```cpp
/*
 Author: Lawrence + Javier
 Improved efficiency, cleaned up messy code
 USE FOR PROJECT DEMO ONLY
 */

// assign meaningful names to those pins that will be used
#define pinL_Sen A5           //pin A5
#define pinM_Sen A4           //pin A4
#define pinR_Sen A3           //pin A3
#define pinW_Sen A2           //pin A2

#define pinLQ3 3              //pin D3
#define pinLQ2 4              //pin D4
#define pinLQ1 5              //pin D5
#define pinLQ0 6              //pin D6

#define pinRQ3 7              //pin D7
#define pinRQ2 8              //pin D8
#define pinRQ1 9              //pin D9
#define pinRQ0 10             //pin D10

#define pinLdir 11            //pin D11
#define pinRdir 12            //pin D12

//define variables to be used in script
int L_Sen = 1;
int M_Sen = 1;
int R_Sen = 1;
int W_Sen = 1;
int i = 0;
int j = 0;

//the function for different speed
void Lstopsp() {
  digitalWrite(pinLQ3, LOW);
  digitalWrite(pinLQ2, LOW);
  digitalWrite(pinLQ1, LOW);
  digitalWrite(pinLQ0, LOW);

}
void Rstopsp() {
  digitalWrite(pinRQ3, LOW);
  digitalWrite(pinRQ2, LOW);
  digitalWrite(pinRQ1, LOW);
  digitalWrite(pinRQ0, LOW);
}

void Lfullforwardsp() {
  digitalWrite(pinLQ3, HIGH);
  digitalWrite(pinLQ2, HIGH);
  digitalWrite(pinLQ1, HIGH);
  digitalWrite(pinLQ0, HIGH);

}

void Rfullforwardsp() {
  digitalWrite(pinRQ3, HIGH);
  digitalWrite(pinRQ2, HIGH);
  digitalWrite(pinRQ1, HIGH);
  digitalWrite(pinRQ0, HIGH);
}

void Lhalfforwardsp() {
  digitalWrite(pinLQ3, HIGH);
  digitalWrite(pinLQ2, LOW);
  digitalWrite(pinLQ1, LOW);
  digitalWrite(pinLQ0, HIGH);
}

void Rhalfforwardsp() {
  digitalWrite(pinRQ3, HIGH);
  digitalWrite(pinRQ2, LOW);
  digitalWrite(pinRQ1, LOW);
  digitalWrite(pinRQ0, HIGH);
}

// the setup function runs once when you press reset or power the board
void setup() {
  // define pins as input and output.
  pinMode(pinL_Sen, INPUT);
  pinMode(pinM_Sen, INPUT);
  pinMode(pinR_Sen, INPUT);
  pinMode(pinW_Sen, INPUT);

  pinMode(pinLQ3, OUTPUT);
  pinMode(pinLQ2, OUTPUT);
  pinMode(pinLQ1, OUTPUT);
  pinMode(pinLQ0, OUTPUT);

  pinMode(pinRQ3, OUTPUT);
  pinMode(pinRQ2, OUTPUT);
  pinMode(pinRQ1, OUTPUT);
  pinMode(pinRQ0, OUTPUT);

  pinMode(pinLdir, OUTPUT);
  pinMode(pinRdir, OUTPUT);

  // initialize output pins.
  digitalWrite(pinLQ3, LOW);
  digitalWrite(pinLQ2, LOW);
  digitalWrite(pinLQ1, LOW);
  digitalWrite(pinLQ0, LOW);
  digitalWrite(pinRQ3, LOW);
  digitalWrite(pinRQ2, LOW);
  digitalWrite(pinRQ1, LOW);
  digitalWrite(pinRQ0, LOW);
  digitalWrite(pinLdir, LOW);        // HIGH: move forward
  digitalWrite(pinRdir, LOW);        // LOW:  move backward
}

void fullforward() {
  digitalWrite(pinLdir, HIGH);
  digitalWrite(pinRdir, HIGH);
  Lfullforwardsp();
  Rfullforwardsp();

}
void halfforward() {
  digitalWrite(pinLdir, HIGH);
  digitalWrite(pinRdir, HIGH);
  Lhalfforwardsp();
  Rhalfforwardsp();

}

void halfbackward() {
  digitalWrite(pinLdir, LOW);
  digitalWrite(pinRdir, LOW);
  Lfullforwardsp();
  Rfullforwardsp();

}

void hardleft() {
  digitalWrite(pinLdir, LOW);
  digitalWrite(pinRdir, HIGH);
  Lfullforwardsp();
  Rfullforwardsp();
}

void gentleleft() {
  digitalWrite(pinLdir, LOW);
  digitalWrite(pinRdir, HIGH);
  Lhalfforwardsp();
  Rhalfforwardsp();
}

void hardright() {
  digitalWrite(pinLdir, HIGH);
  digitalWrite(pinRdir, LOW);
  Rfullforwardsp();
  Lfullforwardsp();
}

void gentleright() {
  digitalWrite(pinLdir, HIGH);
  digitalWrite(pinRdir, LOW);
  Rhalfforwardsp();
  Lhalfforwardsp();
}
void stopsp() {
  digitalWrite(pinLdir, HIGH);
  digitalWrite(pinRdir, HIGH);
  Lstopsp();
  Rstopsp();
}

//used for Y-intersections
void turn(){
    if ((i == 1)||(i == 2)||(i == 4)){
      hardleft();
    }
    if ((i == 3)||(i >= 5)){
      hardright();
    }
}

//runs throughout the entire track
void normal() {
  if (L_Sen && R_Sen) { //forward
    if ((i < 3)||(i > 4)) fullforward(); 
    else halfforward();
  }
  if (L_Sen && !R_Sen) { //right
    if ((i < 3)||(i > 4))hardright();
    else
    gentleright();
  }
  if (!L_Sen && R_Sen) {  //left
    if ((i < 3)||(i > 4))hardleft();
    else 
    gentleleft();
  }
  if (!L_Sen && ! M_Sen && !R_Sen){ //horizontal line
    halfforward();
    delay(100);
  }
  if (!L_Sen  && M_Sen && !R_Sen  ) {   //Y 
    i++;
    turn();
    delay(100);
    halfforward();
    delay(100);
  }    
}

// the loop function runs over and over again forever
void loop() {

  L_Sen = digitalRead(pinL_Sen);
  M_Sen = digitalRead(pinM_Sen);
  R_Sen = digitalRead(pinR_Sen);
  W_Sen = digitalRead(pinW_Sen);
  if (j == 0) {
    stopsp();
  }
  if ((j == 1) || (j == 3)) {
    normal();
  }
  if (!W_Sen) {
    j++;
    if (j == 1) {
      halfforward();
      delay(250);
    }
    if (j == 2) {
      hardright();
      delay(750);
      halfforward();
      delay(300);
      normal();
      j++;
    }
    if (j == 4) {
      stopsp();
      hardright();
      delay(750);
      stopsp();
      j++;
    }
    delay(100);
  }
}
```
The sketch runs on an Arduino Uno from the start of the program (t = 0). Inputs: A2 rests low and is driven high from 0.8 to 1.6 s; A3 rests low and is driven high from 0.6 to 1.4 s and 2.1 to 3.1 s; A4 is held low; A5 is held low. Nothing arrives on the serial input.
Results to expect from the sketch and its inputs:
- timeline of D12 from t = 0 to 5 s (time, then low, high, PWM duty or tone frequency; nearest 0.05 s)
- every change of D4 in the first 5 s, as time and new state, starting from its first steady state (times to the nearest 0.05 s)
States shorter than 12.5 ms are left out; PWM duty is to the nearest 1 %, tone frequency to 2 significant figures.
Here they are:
0 s high; 0.45 s low; 1.2 s high; 1.8 s low; 2.55 s high
0 s low; 0.45 s high; 1.2 s low; 1.8 s high; 2.55 s low
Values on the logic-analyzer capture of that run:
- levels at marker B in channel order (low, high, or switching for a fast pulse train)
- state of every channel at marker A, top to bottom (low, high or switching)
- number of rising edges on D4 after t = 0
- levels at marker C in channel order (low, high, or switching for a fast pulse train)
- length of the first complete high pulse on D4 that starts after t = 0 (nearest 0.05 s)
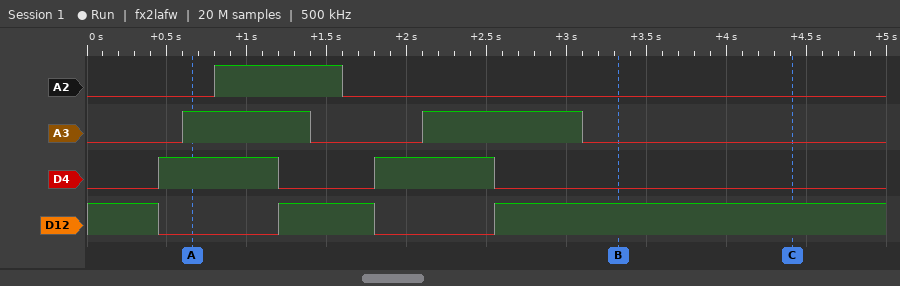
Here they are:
A2 low, A3 low, D4 low, D12 high
A2 low, A3 high, D4 high, D12 low
2
A2 low, A3 low, D4 low, D12 high
0.75 s
